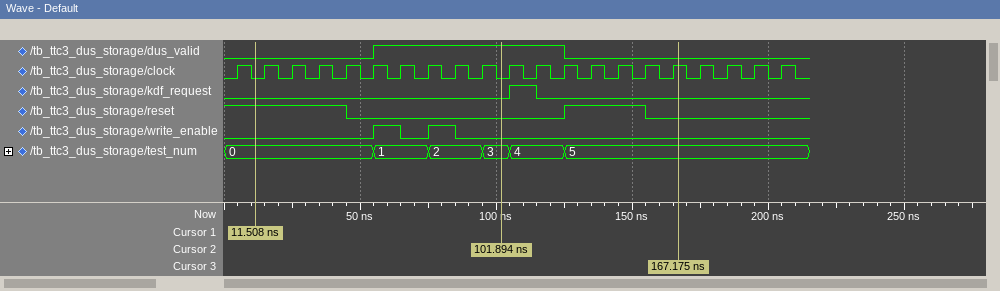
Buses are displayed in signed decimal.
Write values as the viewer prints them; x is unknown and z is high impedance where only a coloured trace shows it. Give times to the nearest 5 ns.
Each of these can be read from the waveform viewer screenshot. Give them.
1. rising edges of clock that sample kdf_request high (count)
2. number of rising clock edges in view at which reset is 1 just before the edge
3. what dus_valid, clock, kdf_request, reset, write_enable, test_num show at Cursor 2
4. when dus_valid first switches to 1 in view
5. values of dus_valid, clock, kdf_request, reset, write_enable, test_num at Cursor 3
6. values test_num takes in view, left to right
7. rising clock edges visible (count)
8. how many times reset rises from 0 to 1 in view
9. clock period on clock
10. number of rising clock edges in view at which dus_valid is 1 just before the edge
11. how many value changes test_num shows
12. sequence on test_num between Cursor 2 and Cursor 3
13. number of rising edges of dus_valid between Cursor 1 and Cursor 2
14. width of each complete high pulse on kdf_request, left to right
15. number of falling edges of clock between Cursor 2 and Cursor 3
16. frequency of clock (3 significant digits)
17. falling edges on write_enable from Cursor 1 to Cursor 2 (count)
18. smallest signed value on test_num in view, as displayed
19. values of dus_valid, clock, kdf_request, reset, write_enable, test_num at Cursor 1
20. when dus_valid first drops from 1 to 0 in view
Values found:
1
8
dus_valid=1, clock=0, kdf_request=0, reset=0, write_enable=0, test_num=3
55 ns
dus_valid=0, clock=1, kdf_request=0, reset=0, write_enable=0, test_num=5
0, 1, 2, 3, 4, 5
21
1
10 ns
7
5
3, 4, 5
1
10 ns
6
100 MHz
2
0
dus_valid=0, clock=0, kdf_request=0, reset=1, write_enable=0, test_num=0
125 ns
